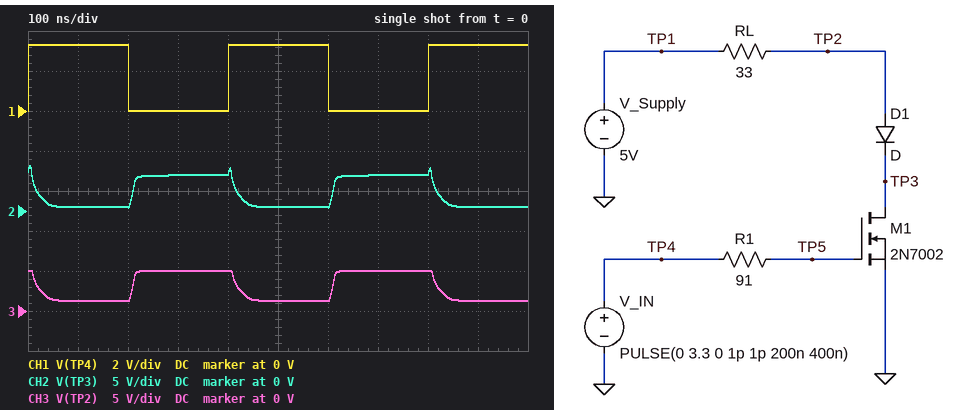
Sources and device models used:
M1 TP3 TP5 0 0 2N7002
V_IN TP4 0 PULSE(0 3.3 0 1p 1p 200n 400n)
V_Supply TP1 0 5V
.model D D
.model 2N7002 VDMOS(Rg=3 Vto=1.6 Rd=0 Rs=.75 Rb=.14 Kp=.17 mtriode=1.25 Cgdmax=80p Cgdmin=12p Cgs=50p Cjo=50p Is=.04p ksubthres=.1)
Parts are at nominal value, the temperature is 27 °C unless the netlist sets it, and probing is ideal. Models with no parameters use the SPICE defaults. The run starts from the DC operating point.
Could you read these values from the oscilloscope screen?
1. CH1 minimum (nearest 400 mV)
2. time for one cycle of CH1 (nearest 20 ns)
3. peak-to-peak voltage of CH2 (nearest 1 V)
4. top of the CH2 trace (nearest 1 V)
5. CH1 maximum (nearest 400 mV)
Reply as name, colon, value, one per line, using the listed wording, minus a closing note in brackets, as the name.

CH1 minimum: 0 V
time for one cycle of CH1: 400 ns
peak-to-peak voltage of CH2: 5 V
top of the CH2 trace: 6 V
CH1 maximum: 3.2 V
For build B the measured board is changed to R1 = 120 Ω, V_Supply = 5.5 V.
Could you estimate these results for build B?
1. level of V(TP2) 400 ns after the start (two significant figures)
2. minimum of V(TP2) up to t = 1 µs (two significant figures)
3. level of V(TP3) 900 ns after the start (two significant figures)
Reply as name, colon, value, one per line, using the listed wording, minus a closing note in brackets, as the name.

level of V(TP2) 400 ns after the start: 5.5 V
minimum of V(TP2) up to t = 1 µs: 1.3 V
level of V(TP3) 900 ns after the start: 580 mV
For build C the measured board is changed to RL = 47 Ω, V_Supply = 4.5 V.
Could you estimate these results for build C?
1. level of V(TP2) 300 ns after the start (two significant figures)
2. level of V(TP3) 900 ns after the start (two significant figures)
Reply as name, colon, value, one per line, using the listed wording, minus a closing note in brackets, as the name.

level of V(TP2) 300 ns after the start: 4.5 V
level of V(TP3) 900 ns after the start: 290 mV
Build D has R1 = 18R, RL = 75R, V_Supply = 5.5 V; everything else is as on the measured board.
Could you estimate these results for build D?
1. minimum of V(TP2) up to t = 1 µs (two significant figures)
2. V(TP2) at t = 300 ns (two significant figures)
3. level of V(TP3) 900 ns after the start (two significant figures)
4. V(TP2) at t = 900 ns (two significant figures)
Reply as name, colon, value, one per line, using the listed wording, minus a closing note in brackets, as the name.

minimum of V(TP2) up to t = 1 µs: 700 mV
V(TP2) at t = 300 ns: 5.5 V
level of V(TP3) 900 ns after the start: 230 mV
V(TP2) at t = 900 ns: 990 mV
